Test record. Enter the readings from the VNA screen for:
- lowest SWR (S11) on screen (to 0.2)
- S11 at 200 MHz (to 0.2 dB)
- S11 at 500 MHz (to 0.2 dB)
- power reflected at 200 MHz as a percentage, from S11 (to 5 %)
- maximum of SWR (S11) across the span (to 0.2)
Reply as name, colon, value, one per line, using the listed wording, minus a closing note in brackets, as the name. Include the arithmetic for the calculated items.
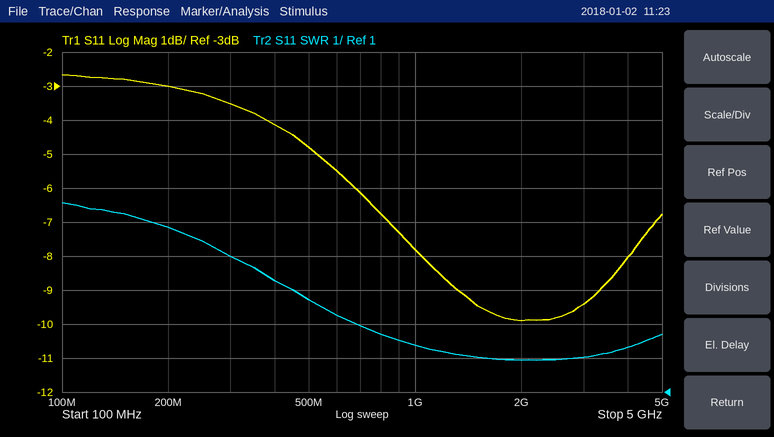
lowest SWR (S11) on screen: 2.0
S11 at 200 MHz: -3.0 dB
S11 at 500 MHz: -4.8 dB
power reflected at 200 MHz as a percentage, from S11: 10^(-3/10) ≈ 50 %
maximum of SWR (S11) across the span: 6.6
